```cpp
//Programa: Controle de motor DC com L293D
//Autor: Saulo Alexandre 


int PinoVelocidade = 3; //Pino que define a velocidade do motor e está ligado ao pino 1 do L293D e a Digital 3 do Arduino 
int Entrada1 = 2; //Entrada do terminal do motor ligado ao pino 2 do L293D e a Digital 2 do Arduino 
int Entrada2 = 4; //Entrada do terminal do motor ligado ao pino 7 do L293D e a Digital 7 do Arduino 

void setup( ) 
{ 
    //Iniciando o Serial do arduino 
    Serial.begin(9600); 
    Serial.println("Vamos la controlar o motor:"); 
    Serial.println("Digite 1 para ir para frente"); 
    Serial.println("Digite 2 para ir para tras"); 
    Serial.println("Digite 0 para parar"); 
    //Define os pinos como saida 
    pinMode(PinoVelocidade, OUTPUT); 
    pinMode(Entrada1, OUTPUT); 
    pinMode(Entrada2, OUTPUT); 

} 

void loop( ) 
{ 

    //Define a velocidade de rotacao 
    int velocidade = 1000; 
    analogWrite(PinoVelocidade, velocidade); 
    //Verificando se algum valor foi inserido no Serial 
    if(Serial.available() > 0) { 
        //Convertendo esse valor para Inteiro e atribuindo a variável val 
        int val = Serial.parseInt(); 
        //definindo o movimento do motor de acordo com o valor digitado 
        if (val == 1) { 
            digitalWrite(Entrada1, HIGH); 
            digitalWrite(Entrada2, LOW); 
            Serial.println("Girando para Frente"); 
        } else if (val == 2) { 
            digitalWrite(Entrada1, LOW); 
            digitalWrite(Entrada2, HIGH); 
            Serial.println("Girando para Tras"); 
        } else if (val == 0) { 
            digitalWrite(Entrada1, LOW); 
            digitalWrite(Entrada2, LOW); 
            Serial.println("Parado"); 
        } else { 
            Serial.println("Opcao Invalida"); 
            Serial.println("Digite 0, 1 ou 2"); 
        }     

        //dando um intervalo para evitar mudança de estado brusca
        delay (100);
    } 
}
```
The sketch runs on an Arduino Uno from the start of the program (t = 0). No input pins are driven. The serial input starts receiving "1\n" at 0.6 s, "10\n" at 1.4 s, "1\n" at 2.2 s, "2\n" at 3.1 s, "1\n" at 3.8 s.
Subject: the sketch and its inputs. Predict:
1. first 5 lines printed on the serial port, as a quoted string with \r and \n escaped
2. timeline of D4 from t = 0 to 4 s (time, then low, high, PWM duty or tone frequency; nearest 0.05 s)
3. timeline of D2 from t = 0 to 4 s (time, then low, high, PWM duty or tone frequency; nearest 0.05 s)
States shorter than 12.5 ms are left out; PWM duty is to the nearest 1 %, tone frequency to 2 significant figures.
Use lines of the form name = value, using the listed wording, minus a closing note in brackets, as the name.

first 5 lines printed on the serial port, as a quoted string with \r and \n escaped = "Vamos la controlar o motor:\r\nDigite 1 para ir para frente\r\nDigite 2 para ir para tras\r\nDigite 0 para parar\r\nGirando para Frente\r\n"
timeline of D4 from t = 0 to 4 s = 0.05 s low; 3.1 s high; 3.8 s low
timeline of D2 from t = 0 to 4 s = 0.05 s low; 0.6 s high; 3.1 s low; 3.8 s high
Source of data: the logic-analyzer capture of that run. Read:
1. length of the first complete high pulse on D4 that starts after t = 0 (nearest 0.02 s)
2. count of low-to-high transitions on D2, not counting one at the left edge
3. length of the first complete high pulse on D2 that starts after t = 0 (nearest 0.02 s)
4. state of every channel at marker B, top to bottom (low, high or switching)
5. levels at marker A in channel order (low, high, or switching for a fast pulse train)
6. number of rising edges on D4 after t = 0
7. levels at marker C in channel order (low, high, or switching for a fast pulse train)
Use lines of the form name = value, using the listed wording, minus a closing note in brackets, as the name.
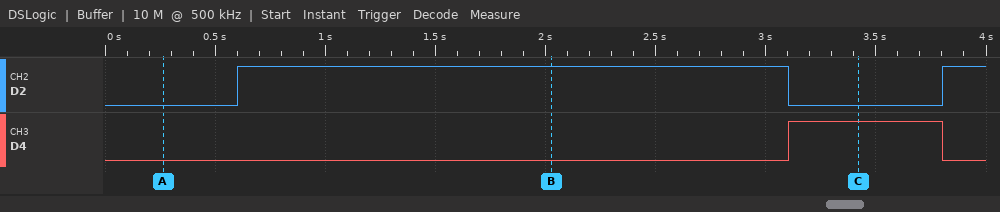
length of the first complete high pulse on D4 that starts after t = 0 = 0.70 s
count of low-to-high transitions on D2, not counting one at the left edge = 2
length of the first complete high pulse on D2 that starts after t = 0 = 2.50 s
state of every channel at marker B, top to bottom = D2 high, D4 low
levels at marker A in channel order = D2 low, D4 low
number of rising edges on D4 after t = 0 = 1
levels at marker C in channel order = D2 low, D4 high
